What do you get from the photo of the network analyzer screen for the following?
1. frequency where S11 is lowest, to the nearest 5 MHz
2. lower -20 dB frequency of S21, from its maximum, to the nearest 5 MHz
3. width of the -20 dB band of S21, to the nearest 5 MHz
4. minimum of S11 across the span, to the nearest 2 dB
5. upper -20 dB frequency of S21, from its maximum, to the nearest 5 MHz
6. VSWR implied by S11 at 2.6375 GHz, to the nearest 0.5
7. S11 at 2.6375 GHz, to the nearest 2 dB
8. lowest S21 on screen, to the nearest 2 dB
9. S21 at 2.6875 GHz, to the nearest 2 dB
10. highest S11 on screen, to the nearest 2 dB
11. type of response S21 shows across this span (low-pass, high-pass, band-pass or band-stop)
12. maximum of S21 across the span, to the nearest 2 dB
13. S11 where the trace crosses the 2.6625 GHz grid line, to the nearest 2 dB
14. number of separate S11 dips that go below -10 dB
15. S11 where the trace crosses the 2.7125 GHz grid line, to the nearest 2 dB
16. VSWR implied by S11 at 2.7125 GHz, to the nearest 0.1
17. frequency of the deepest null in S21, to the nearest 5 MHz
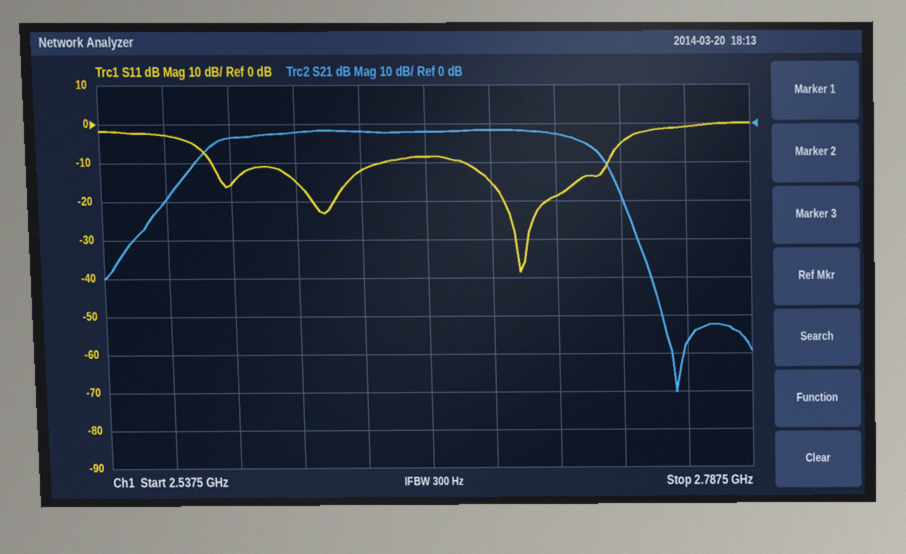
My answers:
2.700 GHz
2.560 GHz
180 MHz
-38 dB
2.740 GHz
1.5
-12 dB
-70 dB
-2 dB
0 dB
band-pass
-2 dB
-8 dB
3
-18 dB
1.3
2.760 GHz
